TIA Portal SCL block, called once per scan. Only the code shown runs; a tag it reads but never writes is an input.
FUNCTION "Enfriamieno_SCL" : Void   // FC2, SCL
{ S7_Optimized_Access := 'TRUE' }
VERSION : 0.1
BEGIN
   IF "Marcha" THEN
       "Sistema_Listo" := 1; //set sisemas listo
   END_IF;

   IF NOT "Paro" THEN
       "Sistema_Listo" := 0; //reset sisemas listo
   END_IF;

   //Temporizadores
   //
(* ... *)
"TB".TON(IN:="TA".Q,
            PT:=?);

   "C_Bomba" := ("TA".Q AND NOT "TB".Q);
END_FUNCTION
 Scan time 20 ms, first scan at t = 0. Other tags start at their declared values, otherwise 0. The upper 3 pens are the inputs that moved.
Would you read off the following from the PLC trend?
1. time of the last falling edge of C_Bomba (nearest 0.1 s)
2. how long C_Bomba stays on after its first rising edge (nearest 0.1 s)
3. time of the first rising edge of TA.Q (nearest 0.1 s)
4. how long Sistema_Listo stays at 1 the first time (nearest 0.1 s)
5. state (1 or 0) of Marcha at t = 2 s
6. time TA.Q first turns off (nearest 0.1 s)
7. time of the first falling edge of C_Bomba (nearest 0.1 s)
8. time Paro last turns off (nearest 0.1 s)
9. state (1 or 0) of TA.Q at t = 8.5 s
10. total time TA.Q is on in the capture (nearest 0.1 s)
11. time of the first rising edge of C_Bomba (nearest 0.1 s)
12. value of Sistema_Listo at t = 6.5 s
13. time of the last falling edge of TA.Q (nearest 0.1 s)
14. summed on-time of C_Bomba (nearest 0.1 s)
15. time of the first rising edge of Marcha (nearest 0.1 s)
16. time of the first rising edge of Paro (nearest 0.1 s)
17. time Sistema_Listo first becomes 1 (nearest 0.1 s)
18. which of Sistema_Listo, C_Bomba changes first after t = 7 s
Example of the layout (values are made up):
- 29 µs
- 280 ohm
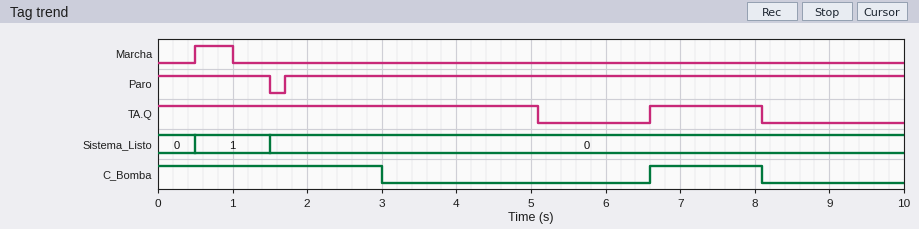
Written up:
- 8.1 s
- 1.5 s
- 6.6 s
- 1.0 s
- 0
- 5.1 s
- 3.0 s
- 1.5 s
- 0
- 6.6 s
- 6.6 s
- 0
- 8.1 s
- 4.5 s
- 0.5 s
- 1.7 s
- 0.5 s
- C_Bomba
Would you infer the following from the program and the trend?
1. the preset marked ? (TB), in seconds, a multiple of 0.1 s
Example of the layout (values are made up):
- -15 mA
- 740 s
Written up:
- 3.0 s
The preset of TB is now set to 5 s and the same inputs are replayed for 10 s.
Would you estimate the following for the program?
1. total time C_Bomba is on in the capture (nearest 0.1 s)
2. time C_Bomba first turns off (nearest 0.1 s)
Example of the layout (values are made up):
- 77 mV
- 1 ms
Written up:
- 6.5 s
- 5.0 s
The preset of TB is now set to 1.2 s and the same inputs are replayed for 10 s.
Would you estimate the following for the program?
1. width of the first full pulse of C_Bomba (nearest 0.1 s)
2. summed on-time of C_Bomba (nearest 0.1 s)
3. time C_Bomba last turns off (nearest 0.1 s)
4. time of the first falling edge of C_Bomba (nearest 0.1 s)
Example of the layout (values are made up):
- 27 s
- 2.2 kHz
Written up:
- 1.2 s
- 2.4 s
- 7.8 s
- 1.2 s
